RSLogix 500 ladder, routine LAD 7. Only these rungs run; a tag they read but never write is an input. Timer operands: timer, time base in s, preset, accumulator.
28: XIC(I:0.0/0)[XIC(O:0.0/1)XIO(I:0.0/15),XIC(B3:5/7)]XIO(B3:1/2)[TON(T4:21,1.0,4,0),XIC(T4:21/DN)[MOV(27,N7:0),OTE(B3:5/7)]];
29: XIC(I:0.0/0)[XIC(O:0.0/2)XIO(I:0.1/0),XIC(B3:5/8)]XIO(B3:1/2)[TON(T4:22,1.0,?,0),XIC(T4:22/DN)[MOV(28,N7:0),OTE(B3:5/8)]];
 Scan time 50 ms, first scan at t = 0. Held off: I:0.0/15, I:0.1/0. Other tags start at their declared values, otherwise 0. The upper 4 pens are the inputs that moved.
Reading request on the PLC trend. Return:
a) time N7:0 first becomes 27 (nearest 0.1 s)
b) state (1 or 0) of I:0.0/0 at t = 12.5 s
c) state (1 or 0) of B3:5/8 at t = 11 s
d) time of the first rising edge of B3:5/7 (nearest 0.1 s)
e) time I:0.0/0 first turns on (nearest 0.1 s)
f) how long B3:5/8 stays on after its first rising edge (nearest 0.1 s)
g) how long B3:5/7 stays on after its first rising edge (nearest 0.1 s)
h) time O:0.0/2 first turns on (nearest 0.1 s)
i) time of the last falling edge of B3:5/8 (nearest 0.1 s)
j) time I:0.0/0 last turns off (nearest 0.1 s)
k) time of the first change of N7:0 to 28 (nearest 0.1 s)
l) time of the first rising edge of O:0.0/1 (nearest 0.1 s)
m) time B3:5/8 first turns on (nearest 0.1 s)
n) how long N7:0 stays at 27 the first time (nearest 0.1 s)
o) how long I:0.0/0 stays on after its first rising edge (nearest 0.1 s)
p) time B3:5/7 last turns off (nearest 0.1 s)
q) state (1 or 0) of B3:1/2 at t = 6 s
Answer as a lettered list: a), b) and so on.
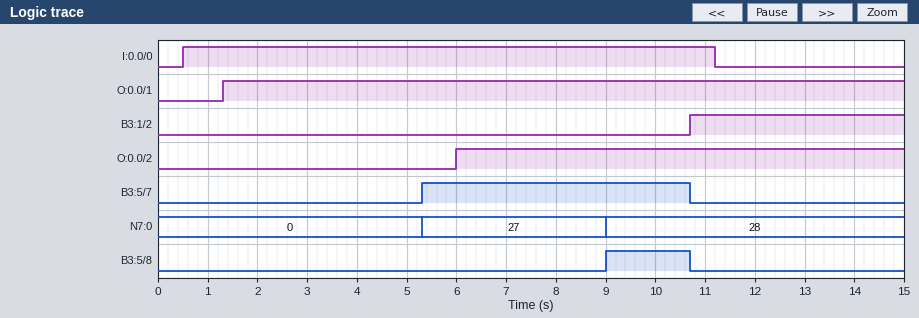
a) 5.3 s
b) 0
c) 0
d) 5.3 s
e) 0.5 s
f) 1.7 s
g) 5.4 s
h) 6.0 s
i) 10.7 s
j) 11.2 s
k) 9.0 s
l) 1.3 s
m) 9.0 s
n) 3.7 s
o) 10.7 s
p) 10.7 s
q) 0
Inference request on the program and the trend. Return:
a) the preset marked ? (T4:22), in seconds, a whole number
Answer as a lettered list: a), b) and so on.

a) 3 s
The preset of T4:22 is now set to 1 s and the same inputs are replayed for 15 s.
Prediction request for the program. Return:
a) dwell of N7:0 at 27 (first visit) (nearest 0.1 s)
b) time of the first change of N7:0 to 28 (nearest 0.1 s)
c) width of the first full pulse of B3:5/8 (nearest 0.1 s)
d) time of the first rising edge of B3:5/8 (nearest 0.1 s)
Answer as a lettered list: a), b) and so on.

a) 1.7 s
b) 7.0 s
c) 3.7 s
d) 7.0 s
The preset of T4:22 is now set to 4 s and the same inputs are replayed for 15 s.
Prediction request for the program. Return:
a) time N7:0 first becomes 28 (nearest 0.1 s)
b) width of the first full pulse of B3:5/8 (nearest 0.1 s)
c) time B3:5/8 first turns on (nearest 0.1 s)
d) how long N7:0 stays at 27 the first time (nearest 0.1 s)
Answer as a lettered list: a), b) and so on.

a) 10.0 s
b) 0.7 s
c) 10.0 s
d) 4.7 s
